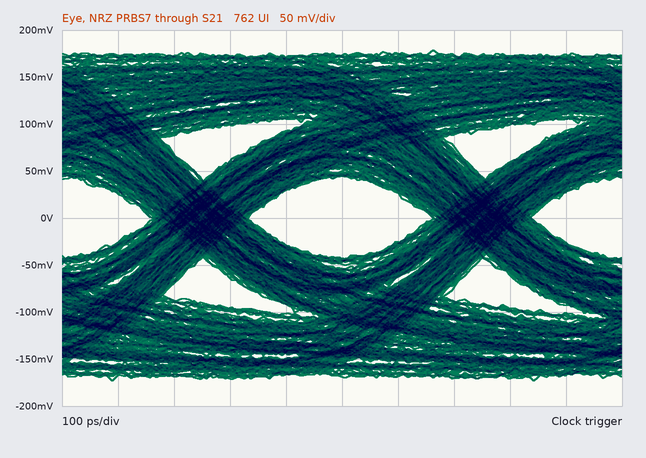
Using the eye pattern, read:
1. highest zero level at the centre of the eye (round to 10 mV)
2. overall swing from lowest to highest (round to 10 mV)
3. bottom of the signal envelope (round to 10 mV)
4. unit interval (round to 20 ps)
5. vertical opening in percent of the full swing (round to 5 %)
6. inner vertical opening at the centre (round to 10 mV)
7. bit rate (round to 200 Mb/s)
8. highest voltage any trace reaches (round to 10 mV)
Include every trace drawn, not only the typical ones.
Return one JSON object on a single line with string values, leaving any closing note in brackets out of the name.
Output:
{"highest zero level at the centre of the eye": "-40 mV", "overall swing from lowest to highest": "350 mV", "bottom of the signal envelope": "-170 mV", "unit interval": "500 ps", "vertical opening in percent of the full swing": "25 %", "inner vertical opening at the centre": "90 mV", "bit rate": "2.0 Gb/s", "highest voltage any trace reaches": "180 mV"}
